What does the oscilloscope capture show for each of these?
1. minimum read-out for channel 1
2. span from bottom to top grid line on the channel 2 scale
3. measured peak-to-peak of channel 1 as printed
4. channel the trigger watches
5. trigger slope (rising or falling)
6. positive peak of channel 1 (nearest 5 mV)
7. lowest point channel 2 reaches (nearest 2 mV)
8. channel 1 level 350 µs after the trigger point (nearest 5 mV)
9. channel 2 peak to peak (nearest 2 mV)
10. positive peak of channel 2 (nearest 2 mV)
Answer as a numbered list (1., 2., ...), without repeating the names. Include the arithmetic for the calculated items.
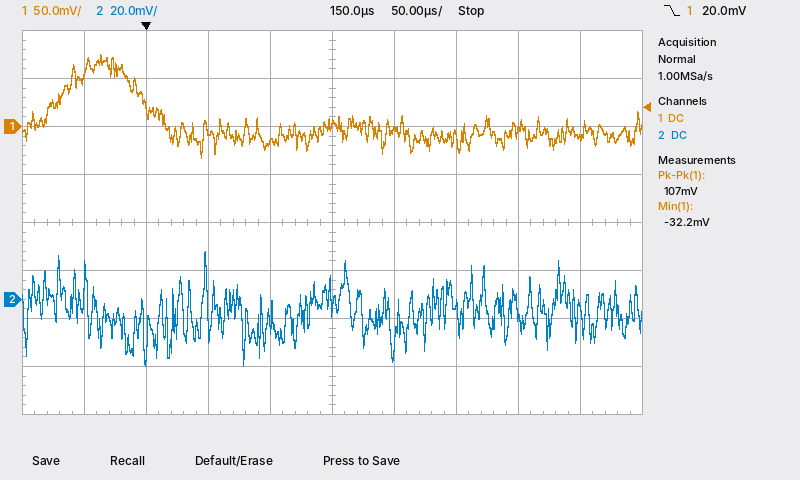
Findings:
1. -32.2 mV
2. 160 mV
3. 107 mV
4. channel 1
5. falling
6. 75 mV
7. -28 mV
8. -10 mV
9. 20 mV − (-28 mV) = 48 mV
10. 20 mV
